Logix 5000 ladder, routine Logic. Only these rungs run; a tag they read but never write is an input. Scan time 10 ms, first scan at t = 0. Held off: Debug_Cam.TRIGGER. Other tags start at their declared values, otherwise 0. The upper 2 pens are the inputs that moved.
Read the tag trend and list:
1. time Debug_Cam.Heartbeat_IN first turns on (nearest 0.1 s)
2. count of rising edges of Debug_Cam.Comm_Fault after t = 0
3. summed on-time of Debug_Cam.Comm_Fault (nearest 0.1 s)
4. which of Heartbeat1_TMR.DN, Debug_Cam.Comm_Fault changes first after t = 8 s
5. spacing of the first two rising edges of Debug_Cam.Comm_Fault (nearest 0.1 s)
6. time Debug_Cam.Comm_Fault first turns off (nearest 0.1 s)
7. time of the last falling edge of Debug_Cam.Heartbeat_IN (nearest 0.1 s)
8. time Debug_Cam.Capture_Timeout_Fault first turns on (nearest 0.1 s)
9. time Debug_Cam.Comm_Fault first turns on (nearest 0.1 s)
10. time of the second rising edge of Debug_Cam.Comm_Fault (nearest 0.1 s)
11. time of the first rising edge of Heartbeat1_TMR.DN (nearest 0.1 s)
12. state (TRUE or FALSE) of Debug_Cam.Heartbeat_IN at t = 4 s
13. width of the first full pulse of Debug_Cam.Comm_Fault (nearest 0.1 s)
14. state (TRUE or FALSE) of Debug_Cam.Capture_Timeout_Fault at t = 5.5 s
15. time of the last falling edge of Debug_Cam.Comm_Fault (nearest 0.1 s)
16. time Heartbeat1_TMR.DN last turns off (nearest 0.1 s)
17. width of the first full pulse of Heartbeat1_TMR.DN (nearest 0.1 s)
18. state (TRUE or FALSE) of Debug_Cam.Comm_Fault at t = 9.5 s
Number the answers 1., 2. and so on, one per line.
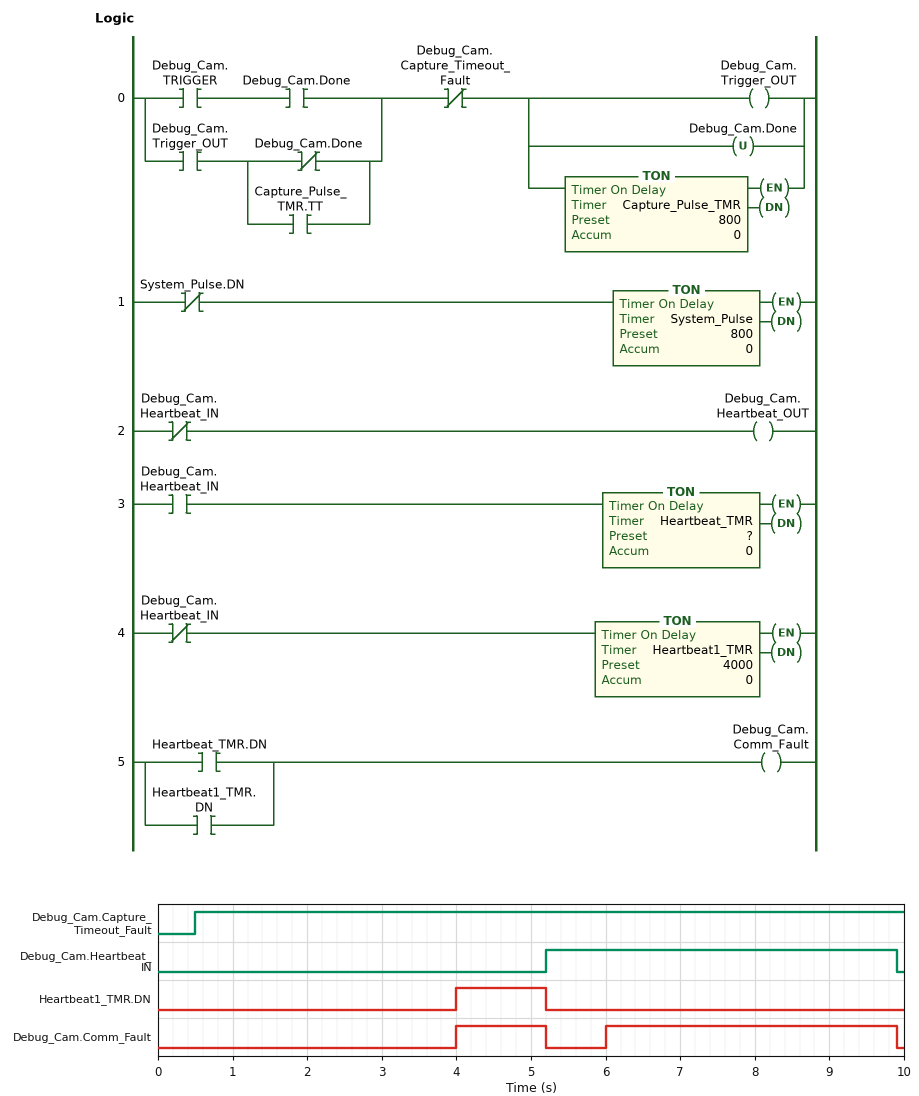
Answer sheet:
1. 5.2 s
2. 2
3. 5.1 s
4. Debug_Cam.Comm_Fault
5. 2.0 s
6. 5.2 s
7. 9.9 s
8. 0.5 s
9. 4.0 s
10. 6.0 s
11. 4.0 s
12. FALSE
13. 1.2 s
14. TRUE
15. 9.9 s
16. 5.2 s
17. 1.2 s
18. TRUE
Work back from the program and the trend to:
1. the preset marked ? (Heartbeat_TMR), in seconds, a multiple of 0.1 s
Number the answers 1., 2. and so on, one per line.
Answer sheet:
1. 0.8 s
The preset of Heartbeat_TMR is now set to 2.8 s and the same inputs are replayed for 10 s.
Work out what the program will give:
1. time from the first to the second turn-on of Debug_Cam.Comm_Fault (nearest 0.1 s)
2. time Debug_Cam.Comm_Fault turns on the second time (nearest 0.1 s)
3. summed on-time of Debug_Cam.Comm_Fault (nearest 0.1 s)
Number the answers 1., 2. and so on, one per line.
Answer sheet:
1. 4.0 s
2. 8.0 s
3. 3.1 s
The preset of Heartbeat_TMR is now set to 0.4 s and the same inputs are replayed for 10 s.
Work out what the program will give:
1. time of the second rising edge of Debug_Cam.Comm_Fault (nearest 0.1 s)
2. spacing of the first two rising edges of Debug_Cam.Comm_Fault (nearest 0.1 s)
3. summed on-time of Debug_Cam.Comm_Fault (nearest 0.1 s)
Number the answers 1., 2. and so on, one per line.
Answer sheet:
1. 5.6 s
2. 1.6 s
3. 5.5 s
